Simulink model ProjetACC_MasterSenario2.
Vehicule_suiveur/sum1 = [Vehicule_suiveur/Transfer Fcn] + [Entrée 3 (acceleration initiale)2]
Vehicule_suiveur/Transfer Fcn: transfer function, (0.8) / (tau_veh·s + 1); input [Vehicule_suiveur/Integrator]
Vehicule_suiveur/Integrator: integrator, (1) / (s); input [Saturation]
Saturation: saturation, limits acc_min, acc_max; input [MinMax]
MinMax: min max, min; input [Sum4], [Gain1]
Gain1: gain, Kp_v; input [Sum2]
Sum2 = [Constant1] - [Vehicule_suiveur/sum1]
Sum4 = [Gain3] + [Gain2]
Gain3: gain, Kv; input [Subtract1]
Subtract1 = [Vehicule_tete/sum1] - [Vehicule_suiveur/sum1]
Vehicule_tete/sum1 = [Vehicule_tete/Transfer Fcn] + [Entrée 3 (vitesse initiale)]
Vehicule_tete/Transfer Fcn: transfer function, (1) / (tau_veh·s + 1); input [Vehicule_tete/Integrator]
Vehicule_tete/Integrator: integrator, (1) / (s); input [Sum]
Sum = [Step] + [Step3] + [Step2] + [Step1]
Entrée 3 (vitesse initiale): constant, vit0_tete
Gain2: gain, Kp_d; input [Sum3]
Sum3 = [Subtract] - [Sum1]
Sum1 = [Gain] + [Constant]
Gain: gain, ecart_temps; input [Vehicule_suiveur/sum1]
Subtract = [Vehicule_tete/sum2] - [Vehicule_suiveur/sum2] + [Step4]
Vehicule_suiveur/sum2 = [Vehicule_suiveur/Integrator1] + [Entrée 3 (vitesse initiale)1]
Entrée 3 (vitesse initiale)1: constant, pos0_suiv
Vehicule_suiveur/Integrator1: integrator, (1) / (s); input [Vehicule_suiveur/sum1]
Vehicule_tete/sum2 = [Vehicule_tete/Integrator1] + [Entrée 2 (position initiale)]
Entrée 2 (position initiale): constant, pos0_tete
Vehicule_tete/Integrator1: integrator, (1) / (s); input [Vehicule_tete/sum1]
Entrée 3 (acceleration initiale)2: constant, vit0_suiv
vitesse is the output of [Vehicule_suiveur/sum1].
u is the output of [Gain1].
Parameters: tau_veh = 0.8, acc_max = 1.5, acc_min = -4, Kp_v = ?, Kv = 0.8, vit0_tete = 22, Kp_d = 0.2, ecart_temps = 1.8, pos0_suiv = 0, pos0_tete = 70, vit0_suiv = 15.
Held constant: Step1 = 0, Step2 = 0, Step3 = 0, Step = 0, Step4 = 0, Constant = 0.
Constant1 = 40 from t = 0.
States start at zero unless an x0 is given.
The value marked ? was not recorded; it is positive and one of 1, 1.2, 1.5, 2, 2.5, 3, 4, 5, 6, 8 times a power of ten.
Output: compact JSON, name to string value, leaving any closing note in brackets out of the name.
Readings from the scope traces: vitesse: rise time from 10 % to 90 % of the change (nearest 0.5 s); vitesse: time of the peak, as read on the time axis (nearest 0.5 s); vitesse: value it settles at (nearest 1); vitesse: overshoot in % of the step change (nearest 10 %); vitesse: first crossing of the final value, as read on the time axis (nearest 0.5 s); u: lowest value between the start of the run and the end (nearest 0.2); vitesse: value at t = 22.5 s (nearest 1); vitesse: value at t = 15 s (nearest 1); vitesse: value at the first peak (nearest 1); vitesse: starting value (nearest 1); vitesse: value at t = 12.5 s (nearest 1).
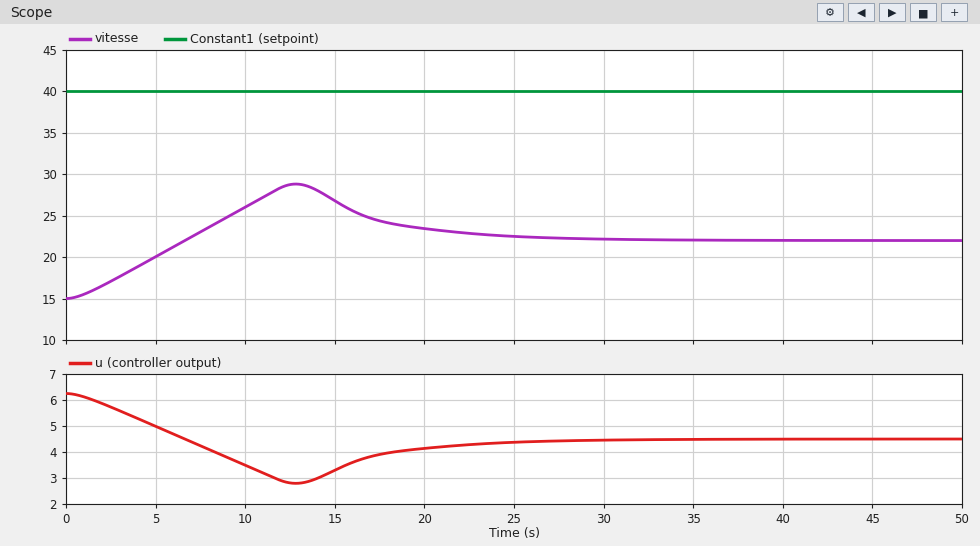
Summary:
{"vitesse: rise time from 10 % to 90 % of the change": "5.0 s", "vitesse: time of the peak, as read on the time axis": "13.0 s", "vitesse: value it settles at": "22", "vitesse: overshoot in % of the step change": "100 %", "vitesse: first crossing of the final value, as read on the time axis": "6.5 s", "u: lowest value between the start of the run and the end": "2.8", "vitesse: value at t = 22.5 s": "23", "vitesse: value at t = 15 s": "27", "vitesse: value at the first peak": "29", "vitesse: starting value": "15", "vitesse: value at t = 12.5 s": "29"}
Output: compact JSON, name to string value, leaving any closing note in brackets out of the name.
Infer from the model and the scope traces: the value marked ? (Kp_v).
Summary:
{"the value marked ?": "0.25"}
